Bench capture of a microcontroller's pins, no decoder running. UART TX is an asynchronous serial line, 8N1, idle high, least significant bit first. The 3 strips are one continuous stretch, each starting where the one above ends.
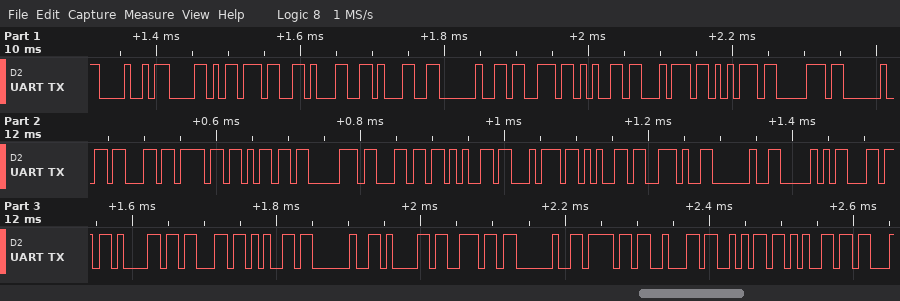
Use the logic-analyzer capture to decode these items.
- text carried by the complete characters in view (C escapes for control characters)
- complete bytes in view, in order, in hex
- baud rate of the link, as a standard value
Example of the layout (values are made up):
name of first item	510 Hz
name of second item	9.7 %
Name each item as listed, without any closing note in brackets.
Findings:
text carried by the complete characters in view	"HX711 setup complete. Place an obje"
complete bytes in view, in order, in hex	48 58 37 31 31 20 73 65 74 75 70 20 63 6F 6D 70 6C 65 74 65 2E 20 50 6C 61 63 65 20 61 6E 20 6F 62 6A 65
baud rate of the link, as a standard value	115200 baud
